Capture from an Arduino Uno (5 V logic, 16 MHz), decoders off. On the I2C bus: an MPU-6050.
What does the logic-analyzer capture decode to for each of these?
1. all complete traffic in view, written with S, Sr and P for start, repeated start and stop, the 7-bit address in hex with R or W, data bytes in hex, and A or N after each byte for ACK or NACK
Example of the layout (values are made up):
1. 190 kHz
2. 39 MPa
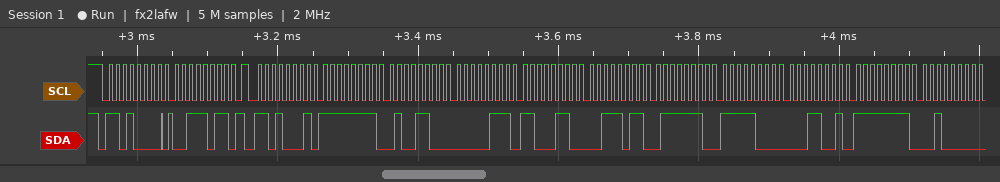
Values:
1. S 68W A 3B A Sr 68R A FF A 4C A 07 A C6 A 3B A 7E A F8 A 19 A FF A 20 A
